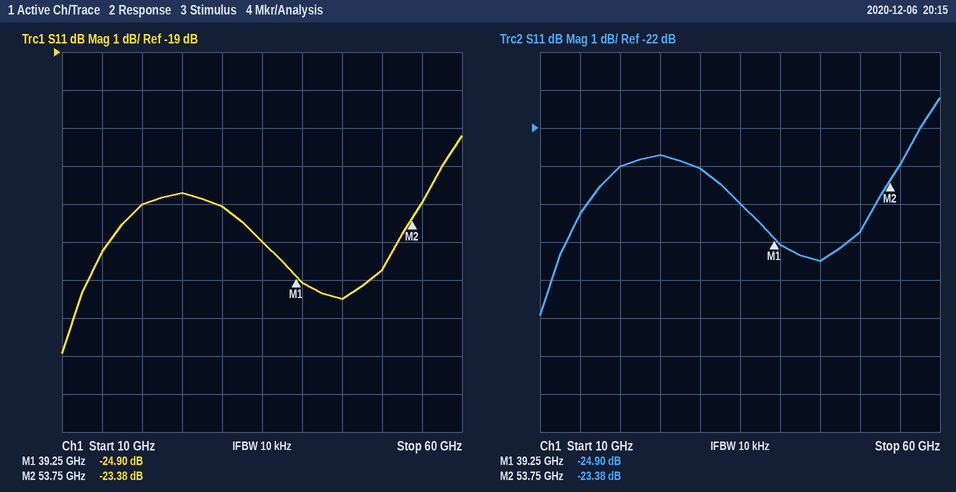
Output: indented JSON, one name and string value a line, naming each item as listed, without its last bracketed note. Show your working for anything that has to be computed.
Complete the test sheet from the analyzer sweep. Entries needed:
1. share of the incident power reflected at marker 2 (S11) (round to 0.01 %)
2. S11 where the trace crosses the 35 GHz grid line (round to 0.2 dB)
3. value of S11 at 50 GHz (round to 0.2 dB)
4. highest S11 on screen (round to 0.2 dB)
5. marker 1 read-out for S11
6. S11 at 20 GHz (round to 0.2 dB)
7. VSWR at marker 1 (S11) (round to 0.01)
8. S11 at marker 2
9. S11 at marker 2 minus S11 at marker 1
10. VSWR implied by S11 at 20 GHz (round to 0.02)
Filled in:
{
  "share of the incident power reflected at marker 2 (S11)": "10^(-23.38/10) ≈ 0.46 %",
  "S11 where the trace crosses the 35 GHz grid line": "-24.0 dB",
  "value of S11 at 50 GHz": "-24.8 dB",
  "highest S11 on screen": "-21.2 dB",
  "marker 1 read-out for S11": "-24.90 dB",
  "S11 at 20 GHz": "-23.0 dB",
  "VSWR at marker 1 (S11)": "(1 + 0.0569)/(1 − 0.0569) ≈ 1.12",
  "S11 at marker 2": "-23.38 dB",
  "S11 at marker 2 minus S11 at marker 1": "-23.38 − (-24.9) = 1.52 dB",
  "VSWR implied by S11 at 20 GHz": "|Γ| = 10^(-23/20) = 0.0708; VSWR = (1 + 0.0708)/(1 − 0.0708) ≈ 1.15, so 1.16 to the nearest 0.02"
}
